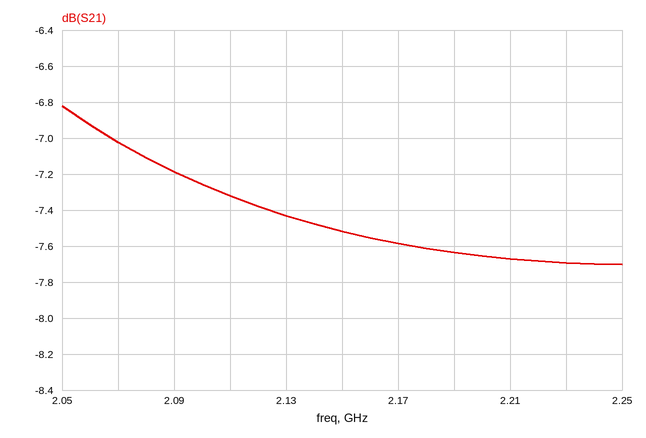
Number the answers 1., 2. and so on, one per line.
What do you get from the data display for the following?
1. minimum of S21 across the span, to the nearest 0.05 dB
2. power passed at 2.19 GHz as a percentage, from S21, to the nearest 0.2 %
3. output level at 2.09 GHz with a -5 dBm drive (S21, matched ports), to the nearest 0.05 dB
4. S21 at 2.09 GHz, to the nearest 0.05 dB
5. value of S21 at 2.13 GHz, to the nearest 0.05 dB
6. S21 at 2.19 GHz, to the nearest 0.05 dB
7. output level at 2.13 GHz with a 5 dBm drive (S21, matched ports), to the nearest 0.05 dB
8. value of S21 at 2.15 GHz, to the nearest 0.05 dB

1. -7.70 dB
2. 17.2 %
3. -12.20 dBm
4. -7.20 dB
5. -7.45 dB
6. -7.65 dB
7. -2.45 dBm
8. -7.50 dB
